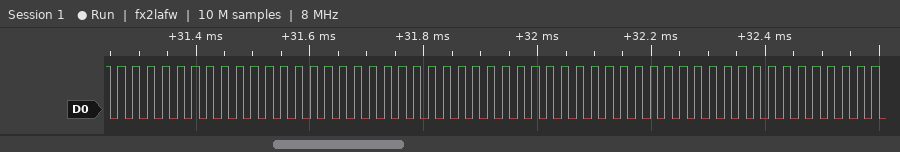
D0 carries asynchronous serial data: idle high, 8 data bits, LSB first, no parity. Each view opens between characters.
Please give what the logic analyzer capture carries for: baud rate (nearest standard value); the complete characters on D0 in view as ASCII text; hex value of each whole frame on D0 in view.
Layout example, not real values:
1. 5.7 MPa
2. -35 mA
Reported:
1. 74880 baud
2. "UUUUUUUUUU"
3. 55, 55, 55, 55, 55, 55, 55, 55, 55, 55
